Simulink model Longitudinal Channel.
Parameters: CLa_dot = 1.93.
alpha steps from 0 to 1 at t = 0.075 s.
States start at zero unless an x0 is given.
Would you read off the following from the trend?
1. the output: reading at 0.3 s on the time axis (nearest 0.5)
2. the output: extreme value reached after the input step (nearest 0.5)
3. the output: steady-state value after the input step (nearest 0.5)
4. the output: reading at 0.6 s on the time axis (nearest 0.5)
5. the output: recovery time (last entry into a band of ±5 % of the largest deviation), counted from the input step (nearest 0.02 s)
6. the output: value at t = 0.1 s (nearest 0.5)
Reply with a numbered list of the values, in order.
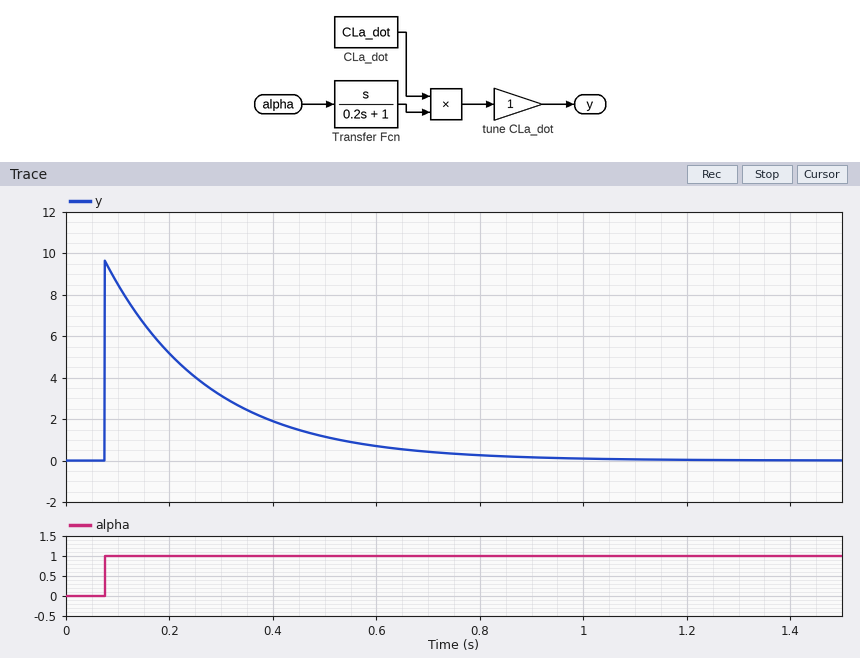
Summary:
1. 3.0
2. 9.5
3. 0.0
4. 0.5
5. 0.60 s
6. 8.5
